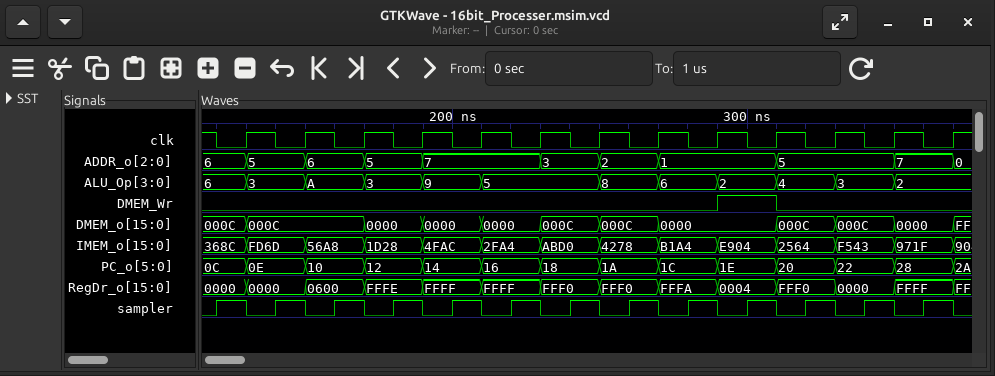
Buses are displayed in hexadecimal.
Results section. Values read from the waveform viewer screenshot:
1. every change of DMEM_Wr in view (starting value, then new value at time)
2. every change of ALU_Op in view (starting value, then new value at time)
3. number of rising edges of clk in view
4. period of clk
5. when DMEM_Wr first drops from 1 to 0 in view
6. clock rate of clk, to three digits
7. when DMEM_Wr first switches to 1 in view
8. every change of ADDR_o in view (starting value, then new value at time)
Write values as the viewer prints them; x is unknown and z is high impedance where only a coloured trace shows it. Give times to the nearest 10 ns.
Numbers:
0, 1 at 290 ns, 0 at 310 ns
6, 3 at 130 ns, A at 150 ns, 3 at 170 ns, 9 at 190 ns, 5 at 210 ns, 8 at 250 ns, 6 at 270 ns, 2 at 290 ns, 4 at 310 ns, 3 at 330 ns, 2 at 350 ns
13
20 ns
310 ns
50.0 MHz
290 ns
6, 5 at 130 ns, 6 at 150 ns, 5 at 170 ns, 7 at 190 ns, 3 at 230 ns, 2 at 250 ns, 1 at 270 ns, 5 at 310 ns, 7 at 350 ns, 0 at 370 ns
